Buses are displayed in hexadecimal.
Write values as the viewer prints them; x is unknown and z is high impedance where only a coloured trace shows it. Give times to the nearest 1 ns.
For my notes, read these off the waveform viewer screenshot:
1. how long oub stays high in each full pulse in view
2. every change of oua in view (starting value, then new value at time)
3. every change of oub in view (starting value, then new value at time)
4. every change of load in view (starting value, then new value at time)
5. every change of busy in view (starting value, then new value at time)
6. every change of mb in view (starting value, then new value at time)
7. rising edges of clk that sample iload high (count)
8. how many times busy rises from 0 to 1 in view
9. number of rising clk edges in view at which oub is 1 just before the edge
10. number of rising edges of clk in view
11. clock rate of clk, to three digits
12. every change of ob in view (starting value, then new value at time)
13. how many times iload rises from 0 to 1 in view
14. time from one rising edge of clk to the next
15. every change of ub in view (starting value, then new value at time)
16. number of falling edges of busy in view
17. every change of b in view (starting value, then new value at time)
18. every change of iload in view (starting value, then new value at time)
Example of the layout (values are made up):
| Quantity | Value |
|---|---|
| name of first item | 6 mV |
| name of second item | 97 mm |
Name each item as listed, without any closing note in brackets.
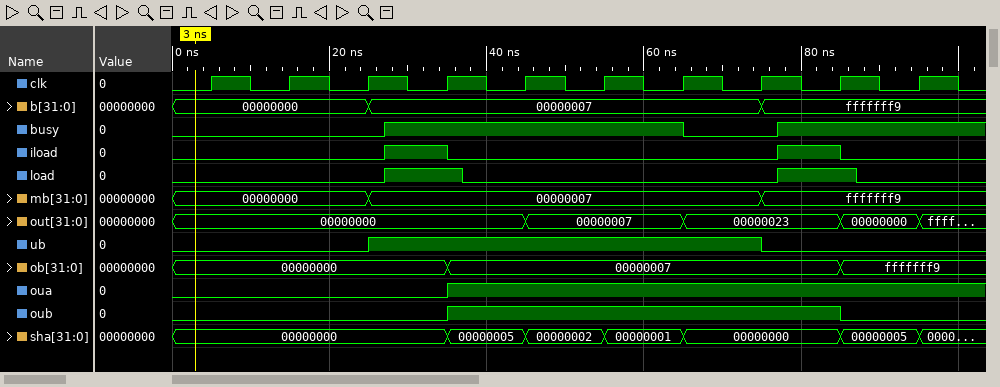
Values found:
| Quantity | Value |
|---|---|
| how long oub stays high in each full pulse in view | 50 ns |
| every change of oua in view | 0, 1 at 35 ns |
| every change of oub in view | 0, 1 at 35 ns, 0 at 85 ns |
| every change of load in view | 0, 1 at 27 ns, 0 at 37 ns, 1 at 77 ns, 0 at 87 ns |
| every change of busy in view | 0, 1 at 27 ns, 0 at 65 ns, 1 at 77 ns |
| every change of mb in view | 00000000, 00000007 at 25 ns, fffffff9 at 75 ns |
| rising edges of clk that sample iload high | 2 |
| how many times busy rises from 0 to 1 in view | 2 |
| number of rising clk edges in view at which oub is 1 just before the edge | 5 |
| number of rising edges of clk in view | 10 |
| clock rate of clk, to three digits | 100 MHz |
| every change of ob in view | 00000000, 00000007 at 35 ns, fffffff9 at 85 ns |
| how many times iload rises from 0 to 1 in view | 2 |
| time from one rising edge of clk to the next | 10 ns |
| every change of ub in view | 0, 1 at 25 ns, 0 at 75 ns |
| number of falling edges of busy in view | 1 |
| every change of b in view | 00000000, 00000007 at 25 ns, fffffff9 at 75 ns |
| every change of iload in view | 0, 1 at 27 ns, 0 at 35 ns, 1 at 77 ns, 0 at 85 ns |
